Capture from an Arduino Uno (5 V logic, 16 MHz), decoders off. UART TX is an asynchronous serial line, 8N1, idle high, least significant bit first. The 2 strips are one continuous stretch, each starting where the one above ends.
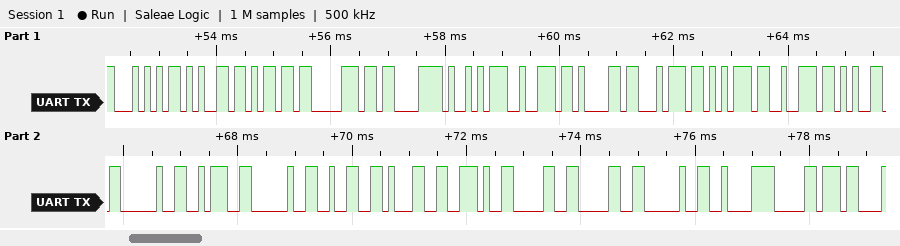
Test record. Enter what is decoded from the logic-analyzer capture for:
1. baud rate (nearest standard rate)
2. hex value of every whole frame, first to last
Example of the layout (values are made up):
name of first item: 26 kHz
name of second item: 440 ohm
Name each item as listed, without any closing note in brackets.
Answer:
baud rate: 9600 baud
hex value of every whole frame, first to last: 54 65 6D 70 C3 A9 72 61 74 75 72 65 20 3A 20 32 31 2E 30 30 20 C2 B0
